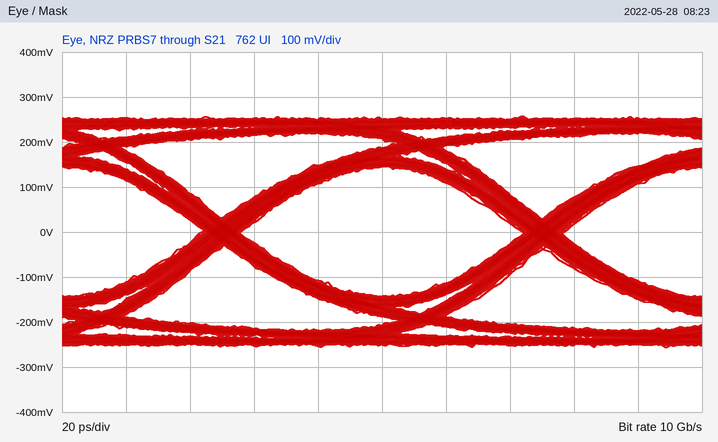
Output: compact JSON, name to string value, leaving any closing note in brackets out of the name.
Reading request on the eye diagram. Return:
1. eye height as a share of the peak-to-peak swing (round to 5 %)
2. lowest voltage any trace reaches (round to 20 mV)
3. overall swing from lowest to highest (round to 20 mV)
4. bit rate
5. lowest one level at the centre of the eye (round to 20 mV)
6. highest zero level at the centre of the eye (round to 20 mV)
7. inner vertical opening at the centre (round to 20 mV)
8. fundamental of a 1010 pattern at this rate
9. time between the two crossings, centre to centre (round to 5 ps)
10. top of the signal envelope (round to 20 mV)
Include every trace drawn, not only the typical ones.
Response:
{"eye height as a share of the peak-to-peak swing": "55 %", "lowest voltage any trace reaches": "-260 mV", "overall swing from lowest to highest": "520 mV", "bit rate": "10 Gb/s", "lowest one level at the centre of the eye": "140 mV", "highest zero level at the centre of the eye": "-140 mV", "inner vertical opening at the centre": "280 mV", "fundamental of a 1010 pattern at this rate": "5 GHz", "time between the two crossings, centre to centre": "100 ps", "top of the signal envelope": "260 mV"}
